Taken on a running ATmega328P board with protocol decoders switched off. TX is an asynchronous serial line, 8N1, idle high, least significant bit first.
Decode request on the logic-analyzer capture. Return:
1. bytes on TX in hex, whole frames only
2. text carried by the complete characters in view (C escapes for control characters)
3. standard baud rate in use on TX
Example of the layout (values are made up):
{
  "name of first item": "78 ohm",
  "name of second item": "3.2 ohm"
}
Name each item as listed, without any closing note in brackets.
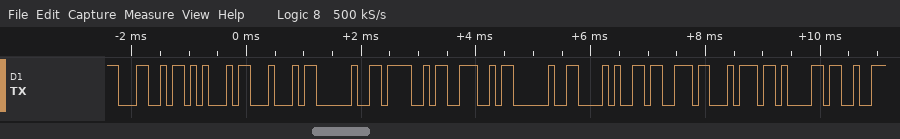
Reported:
{
  "bytes on TX in hex, whole frames only": "4C 45 44 20 4F 4E 20 28 73 74 61",
  "text carried by the complete characters in view": "\"LED ON (sta\"",
  "standard baud rate in use on TX": "9600 baud"
}
